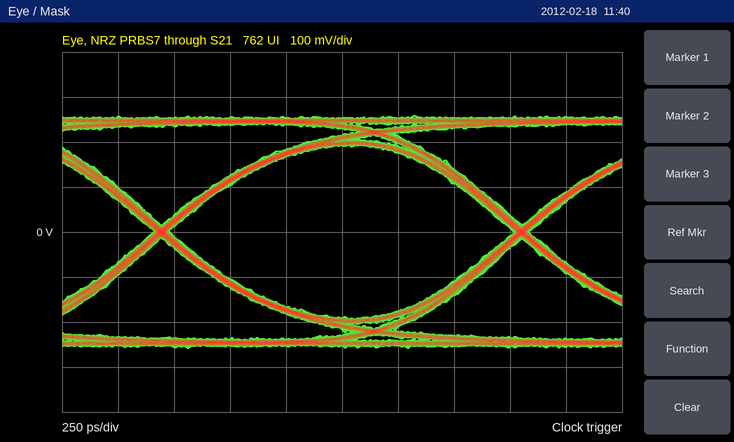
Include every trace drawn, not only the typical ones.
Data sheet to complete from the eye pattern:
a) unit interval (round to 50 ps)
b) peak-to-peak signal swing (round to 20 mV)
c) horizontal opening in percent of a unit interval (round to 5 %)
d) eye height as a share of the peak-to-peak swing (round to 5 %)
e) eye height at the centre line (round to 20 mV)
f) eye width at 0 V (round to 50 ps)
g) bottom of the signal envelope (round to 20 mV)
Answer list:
1.60 ns
520 mV
95 %
75 %
380 mV
1.55 ns
-260 mV
